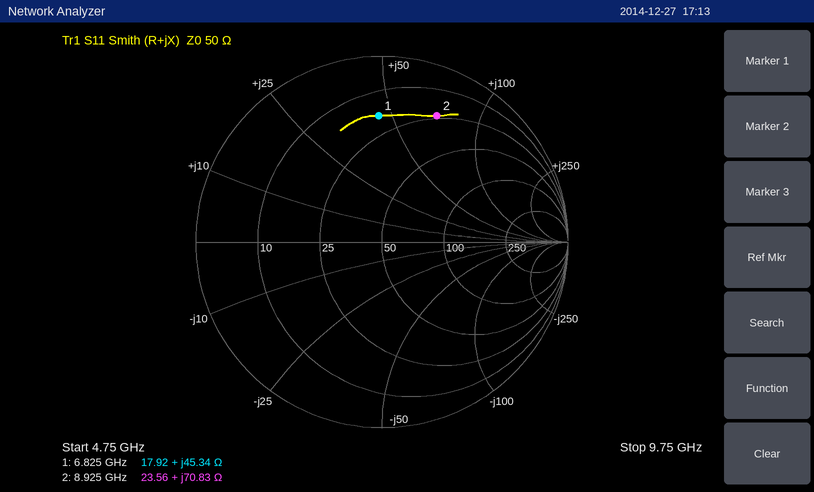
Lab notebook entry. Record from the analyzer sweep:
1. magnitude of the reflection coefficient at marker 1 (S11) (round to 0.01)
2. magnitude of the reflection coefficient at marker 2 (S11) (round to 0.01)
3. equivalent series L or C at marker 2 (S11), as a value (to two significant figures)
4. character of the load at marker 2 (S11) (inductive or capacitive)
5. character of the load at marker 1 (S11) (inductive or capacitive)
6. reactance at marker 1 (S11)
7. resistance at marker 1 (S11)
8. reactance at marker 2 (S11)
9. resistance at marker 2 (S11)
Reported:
0.68
0.74
1.3 nH
inductive
inductive
+45.34 Ω
17.92 Ω
+70.83 Ω
23.56 Ω
